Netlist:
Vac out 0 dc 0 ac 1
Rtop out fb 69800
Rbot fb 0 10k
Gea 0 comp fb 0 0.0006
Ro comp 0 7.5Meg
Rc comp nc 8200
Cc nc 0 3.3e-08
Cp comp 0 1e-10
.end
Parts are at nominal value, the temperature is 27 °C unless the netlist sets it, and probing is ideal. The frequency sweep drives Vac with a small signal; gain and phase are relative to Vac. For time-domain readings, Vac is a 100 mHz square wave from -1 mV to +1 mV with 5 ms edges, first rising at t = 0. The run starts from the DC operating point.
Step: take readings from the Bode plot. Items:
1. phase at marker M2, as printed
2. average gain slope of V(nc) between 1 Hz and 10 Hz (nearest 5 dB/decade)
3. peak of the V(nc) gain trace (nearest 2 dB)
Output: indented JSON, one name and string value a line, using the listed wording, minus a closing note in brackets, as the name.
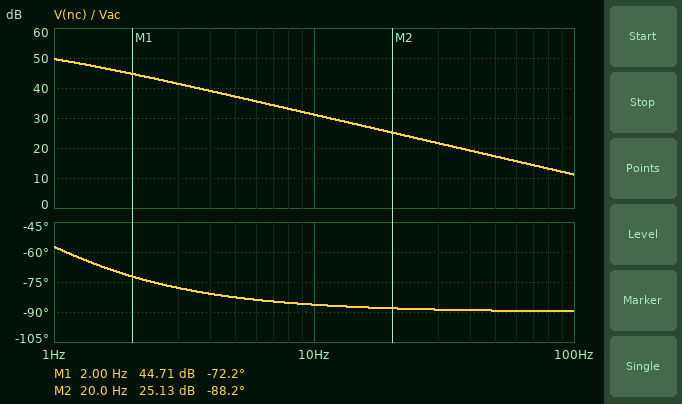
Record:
{
  "phase at marker M2, as printed": "-88.2 deg",
  "average gain slope of V(nc) between 1 Hz and 10 Hz": "-20 dB/decade",
  "peak of the V(nc) gain trace": "50 dB"
}
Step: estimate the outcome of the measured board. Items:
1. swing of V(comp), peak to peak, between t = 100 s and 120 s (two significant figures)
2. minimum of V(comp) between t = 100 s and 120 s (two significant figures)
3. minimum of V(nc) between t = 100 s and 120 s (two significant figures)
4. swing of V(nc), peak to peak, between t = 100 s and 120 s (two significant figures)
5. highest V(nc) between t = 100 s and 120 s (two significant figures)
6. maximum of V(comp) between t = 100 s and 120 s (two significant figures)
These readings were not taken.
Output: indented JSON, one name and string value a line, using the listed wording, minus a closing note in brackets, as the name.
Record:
{
  "swing of V(comp), peak to peak, between t = 100 s and 120 s": "1.1 V",
  "minimum of V(comp) between t = 100 s and 120 s": "-560 mV",
  "minimum of V(nc) between t = 100 s and 120 s": "-560 mV",
  "swing of V(nc), peak to peak, between t = 100 s and 120 s": "1.1 V",
  "highest V(nc) between t = 100 s and 120 s": "560 mV",
  "maximum of V(comp) between t = 100 s and 120 s": "560 mV"
}
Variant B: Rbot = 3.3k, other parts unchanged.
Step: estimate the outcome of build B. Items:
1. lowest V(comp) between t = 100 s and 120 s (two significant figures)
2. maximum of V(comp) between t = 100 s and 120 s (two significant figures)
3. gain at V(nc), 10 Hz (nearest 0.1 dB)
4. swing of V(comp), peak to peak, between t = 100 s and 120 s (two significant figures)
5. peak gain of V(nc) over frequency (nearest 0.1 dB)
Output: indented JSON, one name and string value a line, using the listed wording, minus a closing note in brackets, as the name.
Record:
{
  "lowest V(comp) between t = 100 s and 120 s": "-200 mV",
  "maximum of V(comp) between t = 100 s and 120 s": "200 mV",
  "gain at V(nc), 10 Hz": "22.3 dB",
  "swing of V(comp), peak to peak, between t = 100 s and 120 s": "410 mV",
  "peak gain of V(nc) over frequency": "46.2 dB"
}
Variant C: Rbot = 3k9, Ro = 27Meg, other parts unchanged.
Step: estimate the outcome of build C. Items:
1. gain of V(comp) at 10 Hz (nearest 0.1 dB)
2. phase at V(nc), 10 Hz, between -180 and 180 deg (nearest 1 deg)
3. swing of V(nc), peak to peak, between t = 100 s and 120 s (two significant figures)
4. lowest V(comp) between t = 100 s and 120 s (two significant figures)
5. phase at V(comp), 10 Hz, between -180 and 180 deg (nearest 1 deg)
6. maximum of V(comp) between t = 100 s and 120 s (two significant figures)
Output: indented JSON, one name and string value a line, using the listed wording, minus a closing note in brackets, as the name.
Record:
{
  "gain of V(comp) at 10 Hz": "23.7 dB",
  "phase at V(nc), 10 Hz, between -180 and 180 deg": "-89 deg",
  "swing of V(nc), peak to peak, between t = 100 s and 120 s": "1.7 V",
  "lowest V(comp) between t = 100 s and 120 s": "-850 mV",
  "phase at V(comp), 10 Hz, between -180 and 180 deg": "-88 deg",
  "maximum of V(comp) between t = 100 s and 120 s": "850 mV"
}
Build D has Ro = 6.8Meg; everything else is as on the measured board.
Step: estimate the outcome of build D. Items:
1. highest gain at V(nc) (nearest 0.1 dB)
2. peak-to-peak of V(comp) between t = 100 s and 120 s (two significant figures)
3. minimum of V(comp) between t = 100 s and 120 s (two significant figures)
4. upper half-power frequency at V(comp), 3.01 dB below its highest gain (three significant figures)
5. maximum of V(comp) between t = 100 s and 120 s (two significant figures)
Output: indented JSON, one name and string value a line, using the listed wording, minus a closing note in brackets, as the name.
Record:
{
  "highest gain at V(nc)": "54.2 dB",
  "peak-to-peak of V(comp) between t = 100 s and 120 s": "1.0 V",
  "minimum of V(comp) between t = 100 s and 120 s": "-510 mV",
  "upper half-power frequency at V(comp), 3.01 dB below its highest gain": "706 mHz",
  "maximum of V(comp) between t = 100 s and 120 s": "510 mV"
}
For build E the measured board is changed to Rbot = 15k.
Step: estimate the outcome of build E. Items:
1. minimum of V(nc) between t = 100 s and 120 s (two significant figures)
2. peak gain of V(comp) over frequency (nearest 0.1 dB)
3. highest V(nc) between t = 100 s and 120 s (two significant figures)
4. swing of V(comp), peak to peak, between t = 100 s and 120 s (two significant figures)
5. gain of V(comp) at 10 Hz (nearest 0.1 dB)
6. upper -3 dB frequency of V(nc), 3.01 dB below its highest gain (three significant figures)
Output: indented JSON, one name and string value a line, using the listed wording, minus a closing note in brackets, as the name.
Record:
{
  "minimum of V(nc) between t = 100 s and 120 s": "-800 mV",
  "peak gain of V(comp) over frequency": "58.0 dB",
  "highest V(nc) between t = 100 s and 120 s": "800 mV",
  "swing of V(comp), peak to peak, between t = 100 s and 120 s": "1.6 V",
  "gain of V(comp) at 10 Hz": "34.1 dB",
  "upper -3 dB frequency of V(nc), 3.01 dB below its highest gain": "640 mHz"
}
